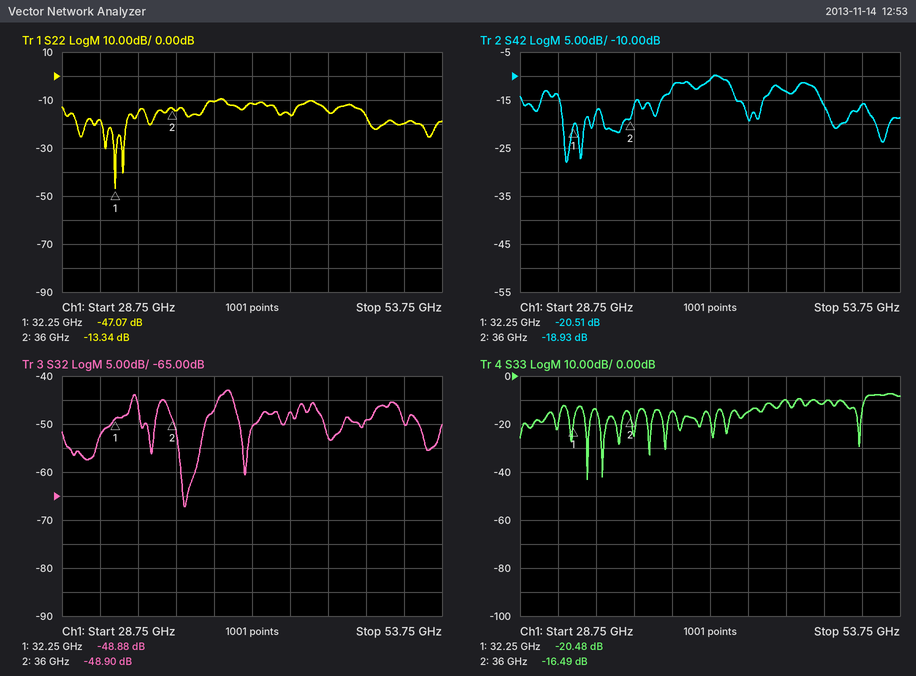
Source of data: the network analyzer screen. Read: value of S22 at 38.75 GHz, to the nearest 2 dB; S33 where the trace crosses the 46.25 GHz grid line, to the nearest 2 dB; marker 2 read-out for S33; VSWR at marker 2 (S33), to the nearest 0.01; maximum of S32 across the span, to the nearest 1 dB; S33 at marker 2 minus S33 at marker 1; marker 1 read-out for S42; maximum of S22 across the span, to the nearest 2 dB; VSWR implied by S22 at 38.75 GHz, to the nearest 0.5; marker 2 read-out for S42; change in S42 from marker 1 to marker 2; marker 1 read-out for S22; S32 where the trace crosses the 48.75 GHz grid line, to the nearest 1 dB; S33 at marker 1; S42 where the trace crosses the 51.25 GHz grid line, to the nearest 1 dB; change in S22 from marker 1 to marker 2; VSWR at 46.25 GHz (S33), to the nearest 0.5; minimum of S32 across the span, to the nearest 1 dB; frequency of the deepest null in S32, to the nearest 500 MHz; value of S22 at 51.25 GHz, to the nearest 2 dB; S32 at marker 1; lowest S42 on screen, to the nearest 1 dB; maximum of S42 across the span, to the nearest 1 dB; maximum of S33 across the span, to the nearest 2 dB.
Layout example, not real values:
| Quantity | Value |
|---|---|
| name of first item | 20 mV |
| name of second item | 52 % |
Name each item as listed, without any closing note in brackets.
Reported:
| Quantity | Value |
|---|---|
| value of S22 at 38.75 GHz, to the nearest 2 dB | -10 dB |
| S33 where the trace crosses the 46.25 GHz grid line, to the nearest 2 dB | -10 dB |
| marker 2 read-out for S33 | -16.49 dB |
| VSWR at marker 2 (S33), to the nearest 0.01 | 1.35 |
| maximum of S32 across the span, to the nearest 1 dB | -43 dB |
| S33 at marker 2 minus S33 at marker 1 | 3.99 dB |
| marker 1 read-out for S42 | -20.51 dB |
| maximum of S22 across the span, to the nearest 2 dB | -10 dB |
| VSWR implied by S22 at 38.75 GHz, to the nearest 0.5 | 2.0 |
| marker 2 read-out for S42 | -18.93 dB |
| change in S42 from marker 1 to marker 2 | 1.58 dB |
| marker 1 read-out for S22 | -47.07 dB |
| S32 where the trace crosses the 48.75 GHz grid line, to the nearest 1 dB | -49 dB |
| S33 at marker 1 | -20.48 dB |
| S42 where the trace crosses the 51.25 GHz grid line, to the nearest 1 dB | -16 dB |
| change in S22 from marker 1 to marker 2 | 33.73 dB |
| VSWR at 46.25 GHz (S33), to the nearest 0.5 | 2.0 |
| minimum of S32 across the span, to the nearest 1 dB | -67 dB |
| frequency of the deepest null in S32, to the nearest 500 MHz | 37.0 GHz |
| value of S22 at 51.25 GHz, to the nearest 2 dB | -20 dB |
| S32 at marker 1 | -48.88 dB |
| lowest S42 on screen, to the nearest 1 dB | -28 dB |
| maximum of S42 across the span, to the nearest 1 dB | -10 dB |
| maximum of S33 across the span, to the nearest 2 dB | -8 dB |
